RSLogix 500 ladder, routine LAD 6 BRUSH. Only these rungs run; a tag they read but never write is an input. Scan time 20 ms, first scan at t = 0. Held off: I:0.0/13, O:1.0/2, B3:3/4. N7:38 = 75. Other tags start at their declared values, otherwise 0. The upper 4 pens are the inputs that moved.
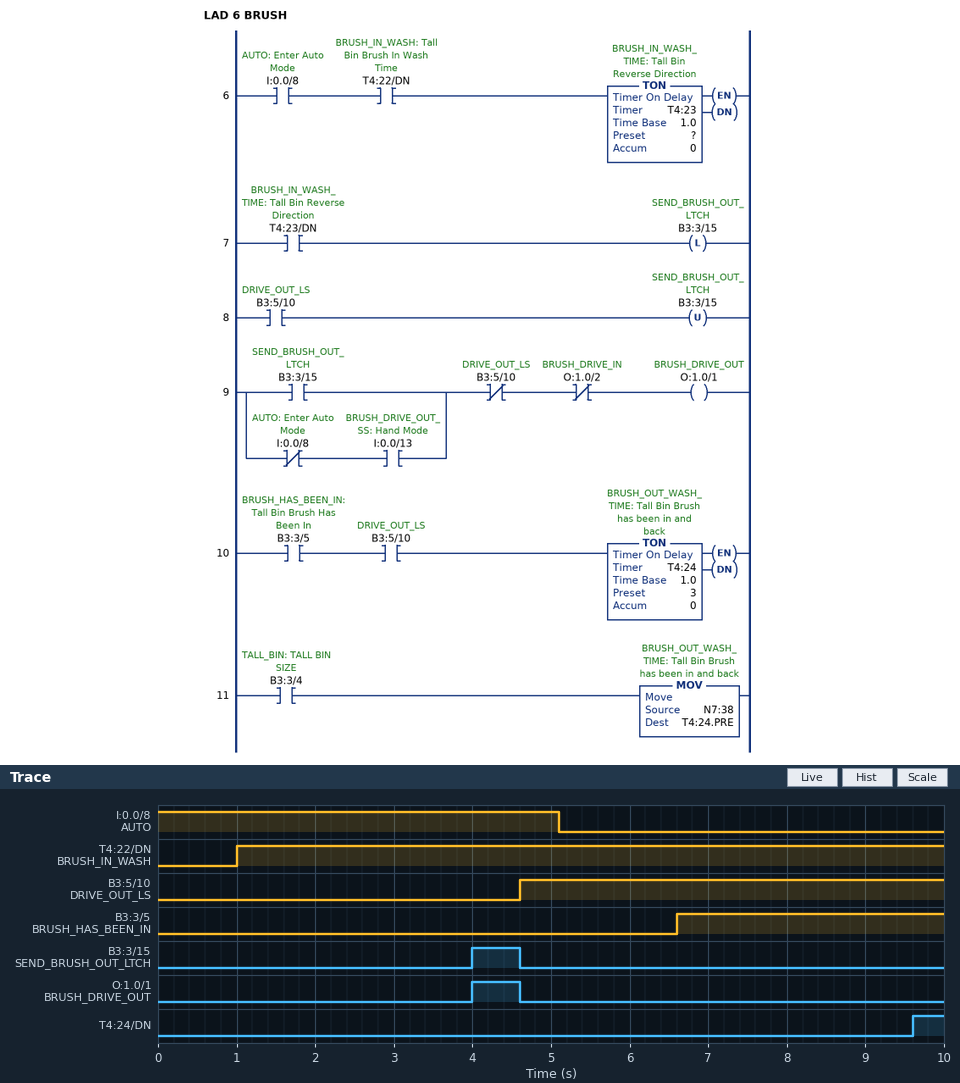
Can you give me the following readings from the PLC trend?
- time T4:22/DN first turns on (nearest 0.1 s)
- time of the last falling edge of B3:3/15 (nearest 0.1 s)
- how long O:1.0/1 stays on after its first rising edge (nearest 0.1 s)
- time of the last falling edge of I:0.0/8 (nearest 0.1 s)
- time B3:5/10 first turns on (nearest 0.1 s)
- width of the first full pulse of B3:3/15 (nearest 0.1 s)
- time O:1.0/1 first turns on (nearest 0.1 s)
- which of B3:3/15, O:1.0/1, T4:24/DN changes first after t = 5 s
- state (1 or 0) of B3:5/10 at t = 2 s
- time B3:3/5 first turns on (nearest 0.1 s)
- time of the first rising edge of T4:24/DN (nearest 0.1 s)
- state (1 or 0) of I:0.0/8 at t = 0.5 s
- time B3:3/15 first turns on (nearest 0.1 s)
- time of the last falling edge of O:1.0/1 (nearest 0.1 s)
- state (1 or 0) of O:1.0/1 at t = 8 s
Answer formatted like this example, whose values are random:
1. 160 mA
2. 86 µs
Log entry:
1. 1.0 s
2. 4.6 s
3. 0.6 s
4. 5.1 s
5. 4.6 s
6. 0.6 s
7. 4.0 s
8. T4:24/DN
9. 0
10. 6.6 s
11. 9.6 s
12. 1
13. 4.0 s
14. 4.6 s
15. 0
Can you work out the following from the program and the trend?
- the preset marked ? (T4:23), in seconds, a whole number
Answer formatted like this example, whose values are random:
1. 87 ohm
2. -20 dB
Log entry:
1. 3 s
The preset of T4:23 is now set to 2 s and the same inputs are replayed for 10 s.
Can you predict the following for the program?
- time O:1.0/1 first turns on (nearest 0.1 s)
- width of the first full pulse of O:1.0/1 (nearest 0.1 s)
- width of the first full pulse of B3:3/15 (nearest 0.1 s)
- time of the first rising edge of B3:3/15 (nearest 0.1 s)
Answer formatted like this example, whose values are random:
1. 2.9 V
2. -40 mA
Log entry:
1. 3.0 s
2. 1.6 s
3. 1.6 s
4. 3.0 s
